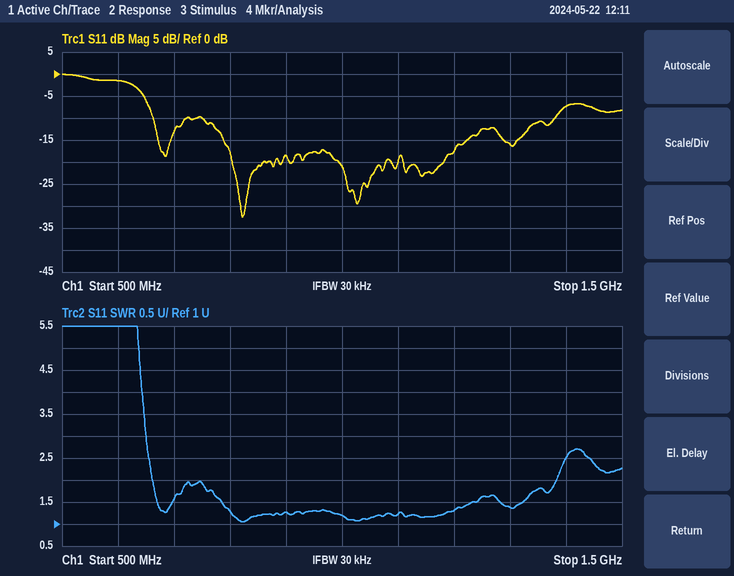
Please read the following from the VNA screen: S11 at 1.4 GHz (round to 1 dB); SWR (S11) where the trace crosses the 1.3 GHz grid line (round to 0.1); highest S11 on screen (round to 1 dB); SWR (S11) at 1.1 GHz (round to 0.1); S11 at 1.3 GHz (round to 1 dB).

-7 dB
1.4
0 dB
1.2
-16 dB
